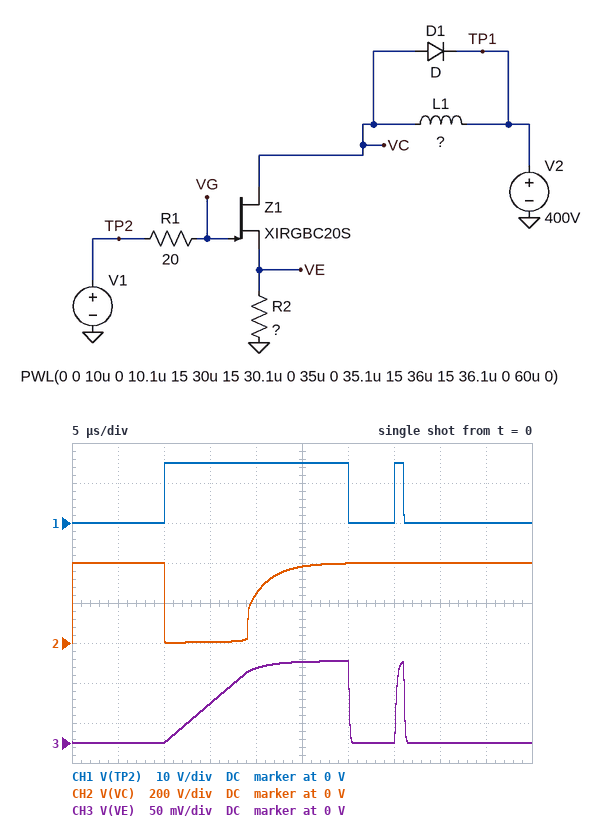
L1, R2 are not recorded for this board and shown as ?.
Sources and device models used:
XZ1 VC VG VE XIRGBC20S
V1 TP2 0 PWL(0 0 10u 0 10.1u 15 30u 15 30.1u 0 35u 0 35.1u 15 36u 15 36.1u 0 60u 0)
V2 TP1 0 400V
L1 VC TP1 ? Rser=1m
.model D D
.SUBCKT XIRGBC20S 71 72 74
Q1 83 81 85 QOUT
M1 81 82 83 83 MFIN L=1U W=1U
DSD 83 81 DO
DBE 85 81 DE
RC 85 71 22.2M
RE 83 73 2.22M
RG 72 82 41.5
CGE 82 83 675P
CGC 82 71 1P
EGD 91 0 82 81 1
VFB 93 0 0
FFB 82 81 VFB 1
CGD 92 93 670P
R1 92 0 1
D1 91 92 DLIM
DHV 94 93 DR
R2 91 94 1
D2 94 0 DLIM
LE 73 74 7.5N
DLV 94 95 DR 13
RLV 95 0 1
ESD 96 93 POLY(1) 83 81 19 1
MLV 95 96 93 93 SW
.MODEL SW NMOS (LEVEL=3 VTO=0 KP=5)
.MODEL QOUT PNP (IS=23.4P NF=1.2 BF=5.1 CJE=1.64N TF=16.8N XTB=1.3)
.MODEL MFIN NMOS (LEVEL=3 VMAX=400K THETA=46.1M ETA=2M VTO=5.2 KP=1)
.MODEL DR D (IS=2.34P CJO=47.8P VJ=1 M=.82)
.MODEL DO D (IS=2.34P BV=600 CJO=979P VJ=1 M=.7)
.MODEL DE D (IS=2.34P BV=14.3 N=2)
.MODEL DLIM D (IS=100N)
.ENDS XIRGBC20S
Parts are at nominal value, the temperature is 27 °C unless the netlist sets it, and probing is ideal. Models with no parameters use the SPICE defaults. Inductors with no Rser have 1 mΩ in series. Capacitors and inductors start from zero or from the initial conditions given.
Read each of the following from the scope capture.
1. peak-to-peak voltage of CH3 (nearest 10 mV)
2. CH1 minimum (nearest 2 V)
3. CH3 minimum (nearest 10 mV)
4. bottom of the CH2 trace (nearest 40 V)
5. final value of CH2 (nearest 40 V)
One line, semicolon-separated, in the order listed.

100 mV; 0 V; 0 V; 0 V; 400 V
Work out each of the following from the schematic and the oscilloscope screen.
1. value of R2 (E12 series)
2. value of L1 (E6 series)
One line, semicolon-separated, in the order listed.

820 µΩ; 33 µH
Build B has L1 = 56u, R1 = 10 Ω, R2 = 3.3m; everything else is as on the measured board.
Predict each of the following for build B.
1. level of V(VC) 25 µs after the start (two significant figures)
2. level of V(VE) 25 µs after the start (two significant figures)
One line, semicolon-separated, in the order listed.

160 V; 350 mV
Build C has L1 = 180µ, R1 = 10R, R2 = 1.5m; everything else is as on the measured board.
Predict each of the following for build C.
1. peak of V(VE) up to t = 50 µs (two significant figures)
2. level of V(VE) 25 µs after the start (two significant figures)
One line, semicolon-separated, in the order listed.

70 mV; 50 mV
